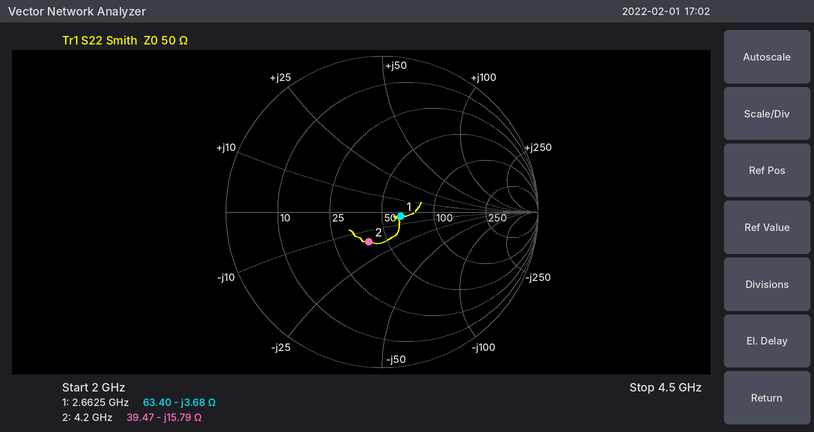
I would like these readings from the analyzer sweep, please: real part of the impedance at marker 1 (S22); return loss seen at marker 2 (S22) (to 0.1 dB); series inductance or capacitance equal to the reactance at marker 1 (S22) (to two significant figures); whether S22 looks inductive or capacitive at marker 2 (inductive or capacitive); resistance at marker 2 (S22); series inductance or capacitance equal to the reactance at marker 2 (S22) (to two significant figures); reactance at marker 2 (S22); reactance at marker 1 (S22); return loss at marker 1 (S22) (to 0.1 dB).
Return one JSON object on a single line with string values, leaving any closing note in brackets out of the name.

{"real part of the impedance at marker 1": "63.40 Ω", "return loss seen at marker 2 (S22)": "13.6 dB", "series inductance or capacitance equal to the reactance at marker 1 (S22)": "16 pF", "whether S22 looks inductive or capacitive at marker 2": "capacitive", "resistance at marker 2": "39.47 Ω", "series inductance or capacitance equal to the reactance at marker 2 (S22)": "2.4 pF", "reactance at marker 2": "-15.79 Ω", "reactance at marker 1": "-3.68 Ω", "return loss at marker 1 (S22)": "18.2 dB"}
